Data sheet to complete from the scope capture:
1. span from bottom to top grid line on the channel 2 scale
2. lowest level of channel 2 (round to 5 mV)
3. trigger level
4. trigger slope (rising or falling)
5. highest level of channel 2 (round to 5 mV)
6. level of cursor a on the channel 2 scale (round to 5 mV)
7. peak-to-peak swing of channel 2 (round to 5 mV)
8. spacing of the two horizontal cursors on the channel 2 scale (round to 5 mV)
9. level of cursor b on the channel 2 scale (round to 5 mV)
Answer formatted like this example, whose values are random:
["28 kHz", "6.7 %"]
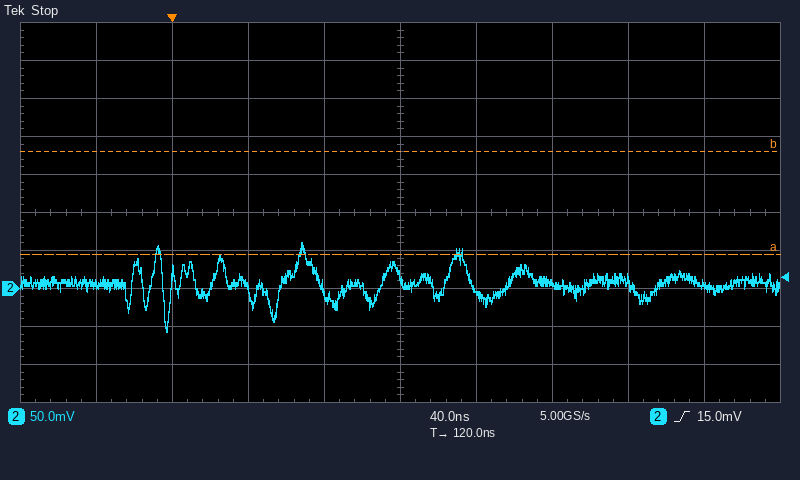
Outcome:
["500 mV", "-55 mV", "15.0 mV", "rising", "60 mV", "45 mV", "115 mV", "135 mV", "180 mV"]
